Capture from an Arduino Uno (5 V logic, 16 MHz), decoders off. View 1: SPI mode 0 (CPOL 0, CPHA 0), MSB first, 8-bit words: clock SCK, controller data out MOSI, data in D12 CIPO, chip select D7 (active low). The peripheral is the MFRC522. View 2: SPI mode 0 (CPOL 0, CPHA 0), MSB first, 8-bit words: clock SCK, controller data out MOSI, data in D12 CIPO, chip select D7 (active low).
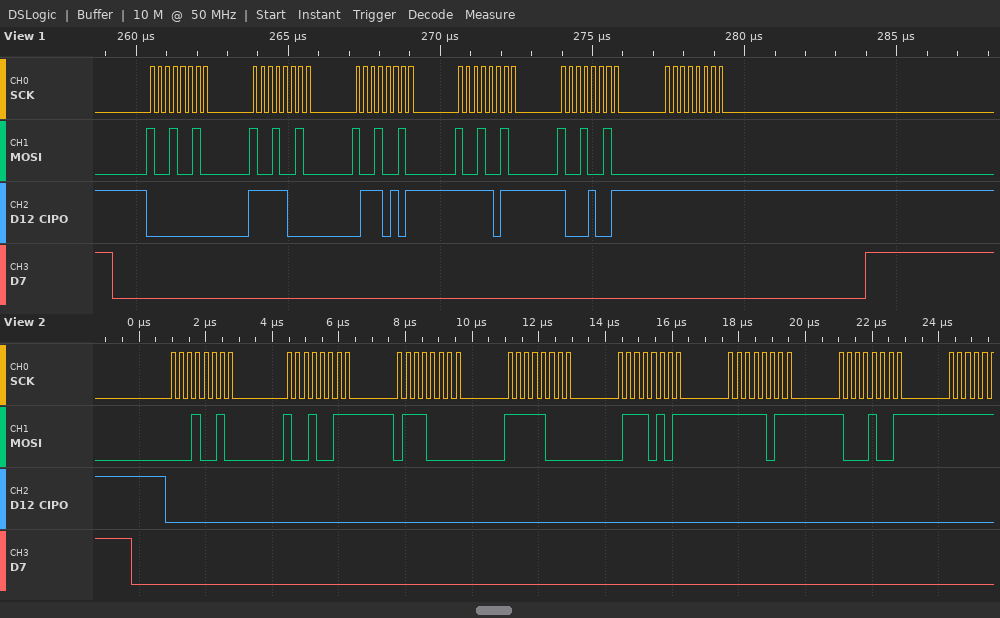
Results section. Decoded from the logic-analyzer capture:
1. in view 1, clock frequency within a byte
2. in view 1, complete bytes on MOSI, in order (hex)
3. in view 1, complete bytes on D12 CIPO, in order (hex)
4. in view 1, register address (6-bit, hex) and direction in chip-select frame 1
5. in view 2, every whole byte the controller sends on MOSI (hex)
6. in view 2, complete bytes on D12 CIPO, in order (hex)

4 MHz
92 92 92 92 92 00
00 F8 75 FB 89 FF
0x09 read
12 93 70 F8 75 FB 89
00 00 00 00 00 00 00
